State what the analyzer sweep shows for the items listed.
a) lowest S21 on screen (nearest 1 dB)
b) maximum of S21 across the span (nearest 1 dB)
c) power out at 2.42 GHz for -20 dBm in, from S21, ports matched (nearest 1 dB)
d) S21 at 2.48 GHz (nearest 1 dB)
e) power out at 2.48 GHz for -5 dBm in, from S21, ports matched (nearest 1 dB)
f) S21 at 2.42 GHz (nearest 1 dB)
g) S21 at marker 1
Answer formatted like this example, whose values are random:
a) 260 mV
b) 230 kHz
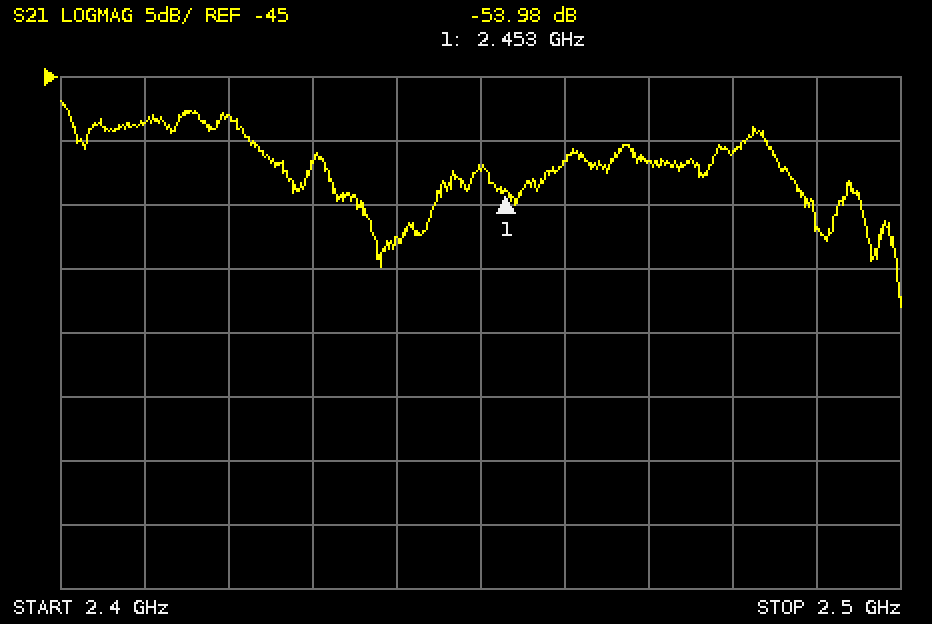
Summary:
a) -63 dB
b) -47 dB
c) -68 dBm
d) -51 dB
e) -56 dBm
f) -48 dB
g) -53.98 dB
